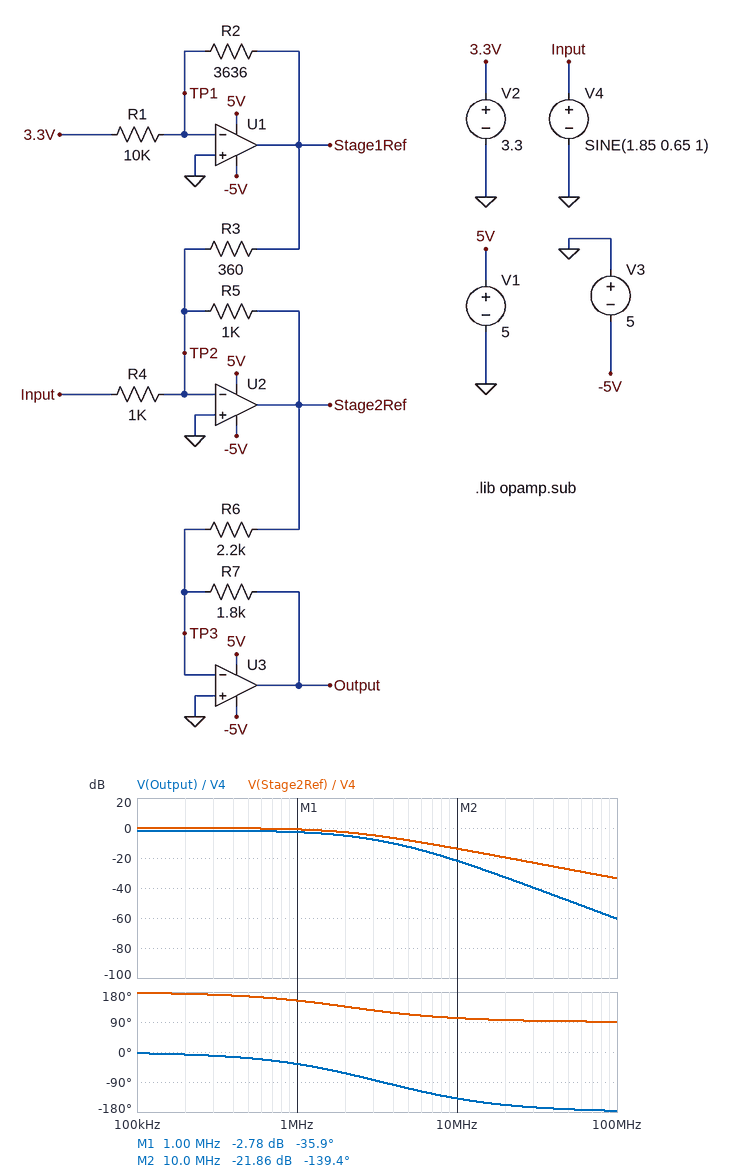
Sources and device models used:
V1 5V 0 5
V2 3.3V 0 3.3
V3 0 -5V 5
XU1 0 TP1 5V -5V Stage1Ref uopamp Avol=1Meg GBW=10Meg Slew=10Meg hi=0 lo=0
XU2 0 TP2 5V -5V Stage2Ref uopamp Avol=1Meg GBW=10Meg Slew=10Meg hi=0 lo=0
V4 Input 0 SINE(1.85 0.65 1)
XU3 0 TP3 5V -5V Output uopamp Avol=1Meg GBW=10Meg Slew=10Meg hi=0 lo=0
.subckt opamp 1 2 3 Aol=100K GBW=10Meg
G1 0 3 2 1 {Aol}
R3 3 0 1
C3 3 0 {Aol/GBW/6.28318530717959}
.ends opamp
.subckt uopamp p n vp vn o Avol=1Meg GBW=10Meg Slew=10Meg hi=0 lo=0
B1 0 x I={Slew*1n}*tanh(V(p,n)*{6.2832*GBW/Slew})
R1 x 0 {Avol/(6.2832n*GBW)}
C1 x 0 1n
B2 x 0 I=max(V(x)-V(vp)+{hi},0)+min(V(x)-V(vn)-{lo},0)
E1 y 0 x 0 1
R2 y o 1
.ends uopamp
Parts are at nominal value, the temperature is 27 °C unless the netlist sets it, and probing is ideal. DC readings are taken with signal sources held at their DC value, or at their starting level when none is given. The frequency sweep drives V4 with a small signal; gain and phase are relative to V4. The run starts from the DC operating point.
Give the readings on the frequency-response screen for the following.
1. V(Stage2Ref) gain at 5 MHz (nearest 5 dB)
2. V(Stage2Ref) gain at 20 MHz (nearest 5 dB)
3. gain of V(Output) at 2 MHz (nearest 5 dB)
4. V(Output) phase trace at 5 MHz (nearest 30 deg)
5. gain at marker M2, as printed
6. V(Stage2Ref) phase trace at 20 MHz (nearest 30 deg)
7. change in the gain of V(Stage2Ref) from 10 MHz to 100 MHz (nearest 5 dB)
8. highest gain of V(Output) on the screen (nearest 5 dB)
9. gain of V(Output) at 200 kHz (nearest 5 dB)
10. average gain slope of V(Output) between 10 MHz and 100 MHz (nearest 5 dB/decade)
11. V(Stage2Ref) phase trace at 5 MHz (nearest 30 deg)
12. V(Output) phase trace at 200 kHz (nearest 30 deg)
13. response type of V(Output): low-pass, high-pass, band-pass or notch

-10 dB
-20 dB
-5 dB
-120 deg
-21.86 dB
90 deg
-20 dB
0 dB
0 dB
-40 dB/decade
120 deg
0 deg
low-pass
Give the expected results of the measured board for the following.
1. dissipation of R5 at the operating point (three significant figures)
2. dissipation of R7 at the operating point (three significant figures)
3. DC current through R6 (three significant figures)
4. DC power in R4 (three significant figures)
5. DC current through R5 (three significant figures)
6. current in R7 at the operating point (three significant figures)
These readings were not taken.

2.20 mW
818 µW
674 µA
3.42 mW
1.48 mA
674 µA
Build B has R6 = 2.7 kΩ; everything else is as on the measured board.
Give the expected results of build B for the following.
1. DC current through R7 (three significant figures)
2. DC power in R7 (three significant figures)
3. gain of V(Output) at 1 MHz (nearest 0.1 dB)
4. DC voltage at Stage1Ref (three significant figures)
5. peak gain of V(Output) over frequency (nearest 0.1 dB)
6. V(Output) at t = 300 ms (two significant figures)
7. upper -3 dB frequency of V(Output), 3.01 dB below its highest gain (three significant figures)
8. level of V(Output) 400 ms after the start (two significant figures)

549 µA
543 µW
-4.5 dB
-1.20 V
-3.5 dB
-580 mV
1.89 MHz
-730 mV
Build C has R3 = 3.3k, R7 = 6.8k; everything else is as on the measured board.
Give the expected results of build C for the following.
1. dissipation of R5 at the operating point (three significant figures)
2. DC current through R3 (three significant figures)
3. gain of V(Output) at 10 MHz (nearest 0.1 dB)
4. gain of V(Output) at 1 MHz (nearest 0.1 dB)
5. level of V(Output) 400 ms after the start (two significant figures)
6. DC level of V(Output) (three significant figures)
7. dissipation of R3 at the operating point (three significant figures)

2.21 mW
364 µA
-10.7 dB
8.9 dB
5.0 V
4.59 V
436 µW
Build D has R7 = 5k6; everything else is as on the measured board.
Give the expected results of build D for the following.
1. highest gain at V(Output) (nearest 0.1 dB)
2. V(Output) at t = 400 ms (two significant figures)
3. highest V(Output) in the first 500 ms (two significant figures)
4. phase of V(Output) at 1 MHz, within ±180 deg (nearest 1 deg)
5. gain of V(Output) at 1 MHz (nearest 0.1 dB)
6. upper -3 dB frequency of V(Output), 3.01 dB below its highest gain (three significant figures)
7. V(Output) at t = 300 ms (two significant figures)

8.1 dB
-2.8 V
-2.1 V
-45 deg
6.7 dB
1.54 MHz
-2.2 V
